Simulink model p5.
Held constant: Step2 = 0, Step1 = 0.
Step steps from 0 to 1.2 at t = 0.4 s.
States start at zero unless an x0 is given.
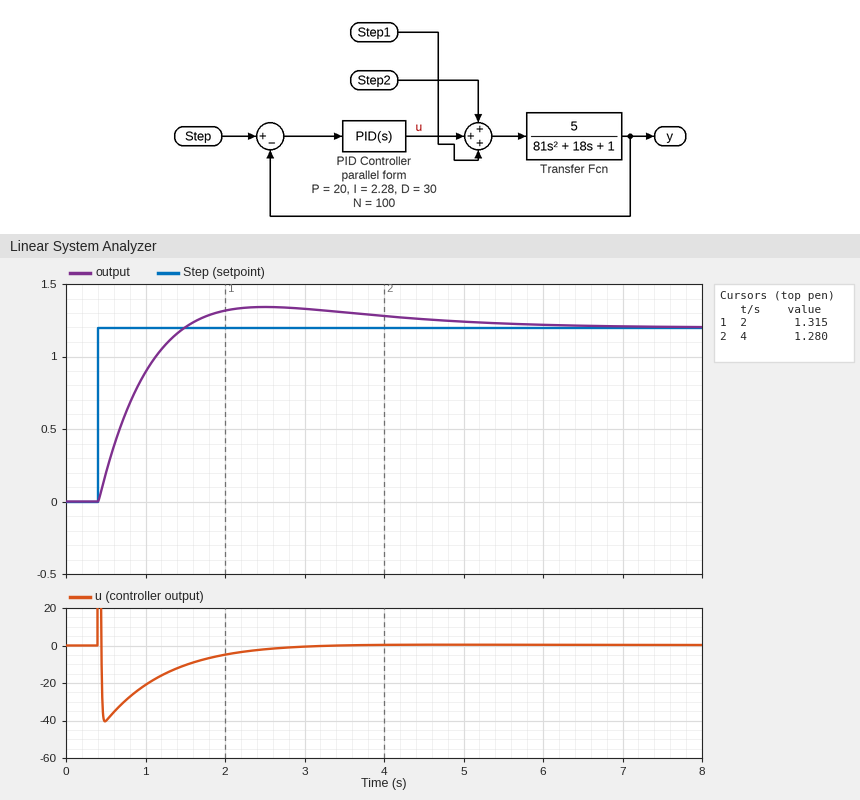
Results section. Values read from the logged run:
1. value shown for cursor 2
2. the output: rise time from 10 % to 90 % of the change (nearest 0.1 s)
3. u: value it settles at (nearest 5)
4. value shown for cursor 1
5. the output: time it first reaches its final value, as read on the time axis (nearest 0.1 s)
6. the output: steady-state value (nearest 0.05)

1.280
0.8 s
0
1.315
1.5 s
1.20
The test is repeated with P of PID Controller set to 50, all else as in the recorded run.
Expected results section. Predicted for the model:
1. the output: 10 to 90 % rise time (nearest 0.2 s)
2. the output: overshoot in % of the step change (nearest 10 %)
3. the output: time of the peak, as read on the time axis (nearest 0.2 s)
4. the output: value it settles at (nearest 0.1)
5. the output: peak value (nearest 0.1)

0.6 s
20 %
1.8 s
1.2
1.5
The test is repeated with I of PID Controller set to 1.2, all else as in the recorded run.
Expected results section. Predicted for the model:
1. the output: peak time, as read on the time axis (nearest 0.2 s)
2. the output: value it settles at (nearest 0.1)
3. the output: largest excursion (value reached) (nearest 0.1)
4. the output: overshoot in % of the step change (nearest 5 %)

2.4 s
1.2
1.3
10 %
